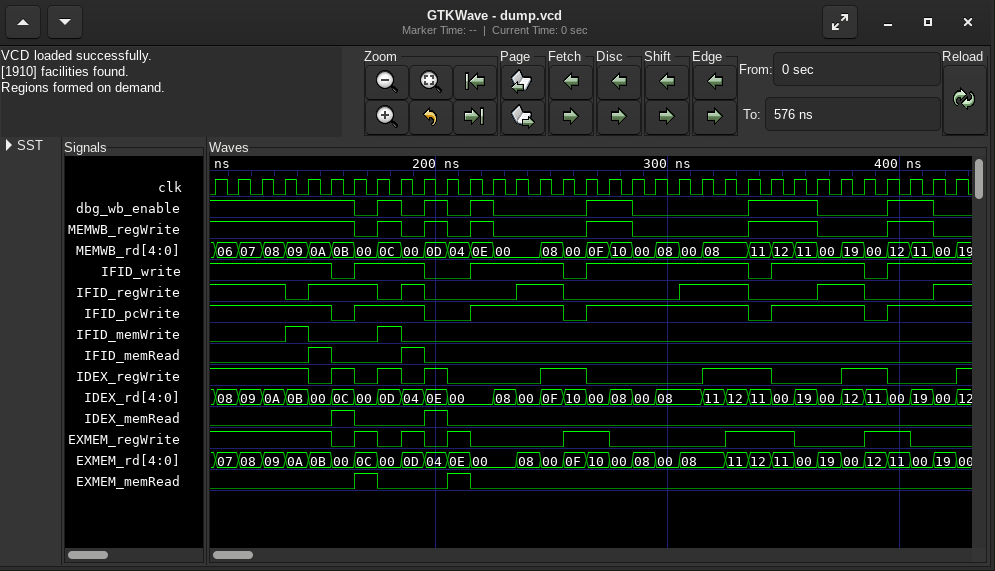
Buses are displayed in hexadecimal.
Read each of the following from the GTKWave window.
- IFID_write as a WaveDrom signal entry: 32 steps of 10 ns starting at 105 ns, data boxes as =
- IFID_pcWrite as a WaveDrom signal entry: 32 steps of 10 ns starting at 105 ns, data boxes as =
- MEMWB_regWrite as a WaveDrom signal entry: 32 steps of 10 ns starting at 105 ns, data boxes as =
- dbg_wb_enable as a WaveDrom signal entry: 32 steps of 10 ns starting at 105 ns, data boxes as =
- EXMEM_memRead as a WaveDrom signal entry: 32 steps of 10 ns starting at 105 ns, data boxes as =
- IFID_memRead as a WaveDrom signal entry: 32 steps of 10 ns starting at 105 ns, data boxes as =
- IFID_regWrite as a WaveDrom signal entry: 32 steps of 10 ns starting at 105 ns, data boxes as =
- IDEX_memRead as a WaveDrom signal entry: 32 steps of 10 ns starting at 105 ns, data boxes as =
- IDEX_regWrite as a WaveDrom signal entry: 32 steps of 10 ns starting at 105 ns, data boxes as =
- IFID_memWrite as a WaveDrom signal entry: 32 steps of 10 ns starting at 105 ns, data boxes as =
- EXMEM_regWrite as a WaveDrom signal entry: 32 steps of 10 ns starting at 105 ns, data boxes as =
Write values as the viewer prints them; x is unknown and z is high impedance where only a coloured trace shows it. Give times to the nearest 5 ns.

{name: 'IFID_write', wave: '1....01..0.1...01......01...01..'}
{name: 'IFID_pcWrite', wave: '1....01..0.1...01......01...01..'}
{name: 'MEMWB_regWrite', wave: '1.....0101010...1.0....1..0..1.0'}
{name: 'dbg_wb_enable', wave: '1.....0101010...1.0....1..0..1.0'}
{name: 'EXMEM_memRead', wave: '0.....10..10....................'}
{name: 'IFID_memRead', wave: '0...10..10......................'}
{name: 'IFID_regWrite', wave: '1..01..010...1.0....1..0..1.0..1'}
{name: 'IDEX_memRead', wave: '0....10..10.....................'}
{name: 'IDEX_regWrite', wave: '1...0101010...1.0....1..0..1.0..'}
{name: 'IFID_memWrite', wave: '0..10..10.......................'}
{name: 'EXMEM_regWrite', wave: '1....0101010...1.0....1..0..1.0.'}
